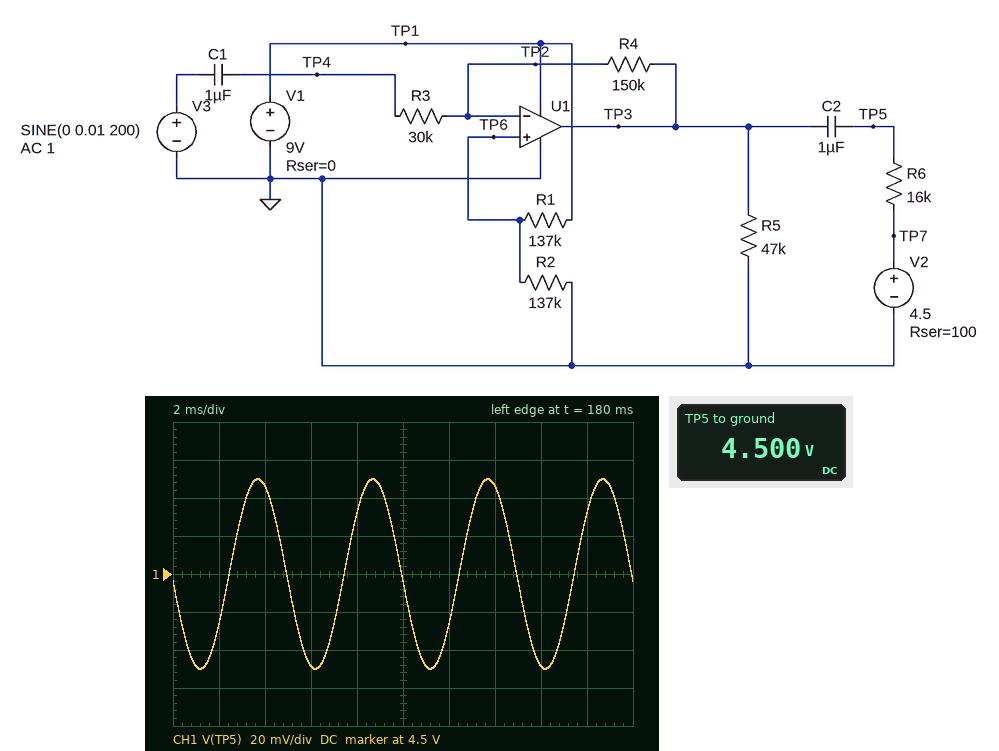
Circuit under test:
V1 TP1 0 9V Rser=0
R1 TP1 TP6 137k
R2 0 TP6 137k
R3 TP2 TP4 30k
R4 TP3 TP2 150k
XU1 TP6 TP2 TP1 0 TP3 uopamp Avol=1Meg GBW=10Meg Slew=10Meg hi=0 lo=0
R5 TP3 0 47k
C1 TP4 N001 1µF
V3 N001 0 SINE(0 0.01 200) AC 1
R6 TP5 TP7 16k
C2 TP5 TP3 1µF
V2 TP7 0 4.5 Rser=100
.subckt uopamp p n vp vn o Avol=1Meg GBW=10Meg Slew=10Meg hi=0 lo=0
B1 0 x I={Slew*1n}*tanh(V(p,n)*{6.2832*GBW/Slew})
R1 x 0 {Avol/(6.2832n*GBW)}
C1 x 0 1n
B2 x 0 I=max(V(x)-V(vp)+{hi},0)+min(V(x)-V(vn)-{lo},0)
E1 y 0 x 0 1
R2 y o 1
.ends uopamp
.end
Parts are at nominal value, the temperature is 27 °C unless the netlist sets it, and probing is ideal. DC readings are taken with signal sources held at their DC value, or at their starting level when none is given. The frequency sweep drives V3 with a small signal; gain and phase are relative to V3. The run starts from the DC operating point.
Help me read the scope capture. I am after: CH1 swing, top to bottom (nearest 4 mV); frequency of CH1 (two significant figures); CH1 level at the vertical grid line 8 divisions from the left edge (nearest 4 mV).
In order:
100 mV
200 Hz
4.452 V
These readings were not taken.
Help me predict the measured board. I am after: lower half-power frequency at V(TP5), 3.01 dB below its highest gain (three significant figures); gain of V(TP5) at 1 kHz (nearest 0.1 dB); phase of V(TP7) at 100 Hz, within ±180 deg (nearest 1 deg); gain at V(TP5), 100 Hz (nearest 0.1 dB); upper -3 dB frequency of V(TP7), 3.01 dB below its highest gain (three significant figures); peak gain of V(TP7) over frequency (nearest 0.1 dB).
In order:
12.0 Hz
14.0 dB
-171 deg
13.9 dB
1.67 MHz
-30.2 dB
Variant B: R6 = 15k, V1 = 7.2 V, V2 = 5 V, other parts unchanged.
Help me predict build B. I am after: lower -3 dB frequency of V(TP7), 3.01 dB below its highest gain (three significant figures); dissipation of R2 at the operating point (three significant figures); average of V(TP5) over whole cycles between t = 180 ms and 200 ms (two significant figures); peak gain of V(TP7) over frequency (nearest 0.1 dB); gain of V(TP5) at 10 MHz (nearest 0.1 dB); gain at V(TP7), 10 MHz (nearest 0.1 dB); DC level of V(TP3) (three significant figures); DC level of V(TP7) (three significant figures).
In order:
12.6 Hz
94.6 µW
5.0 V
-29.6 dB
-1.7 dB
-45.3 dB
3.60 V
5.00 V
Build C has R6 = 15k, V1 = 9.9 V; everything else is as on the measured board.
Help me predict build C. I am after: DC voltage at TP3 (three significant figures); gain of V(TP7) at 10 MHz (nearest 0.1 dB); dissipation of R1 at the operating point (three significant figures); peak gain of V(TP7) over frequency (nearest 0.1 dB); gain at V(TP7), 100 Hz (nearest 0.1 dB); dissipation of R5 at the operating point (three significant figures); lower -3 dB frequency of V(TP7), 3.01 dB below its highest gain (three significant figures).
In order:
4.95 V
-45.3 dB
179 µW
-29.6 dB
-29.7 dB
521 µW
12.6 Hz
